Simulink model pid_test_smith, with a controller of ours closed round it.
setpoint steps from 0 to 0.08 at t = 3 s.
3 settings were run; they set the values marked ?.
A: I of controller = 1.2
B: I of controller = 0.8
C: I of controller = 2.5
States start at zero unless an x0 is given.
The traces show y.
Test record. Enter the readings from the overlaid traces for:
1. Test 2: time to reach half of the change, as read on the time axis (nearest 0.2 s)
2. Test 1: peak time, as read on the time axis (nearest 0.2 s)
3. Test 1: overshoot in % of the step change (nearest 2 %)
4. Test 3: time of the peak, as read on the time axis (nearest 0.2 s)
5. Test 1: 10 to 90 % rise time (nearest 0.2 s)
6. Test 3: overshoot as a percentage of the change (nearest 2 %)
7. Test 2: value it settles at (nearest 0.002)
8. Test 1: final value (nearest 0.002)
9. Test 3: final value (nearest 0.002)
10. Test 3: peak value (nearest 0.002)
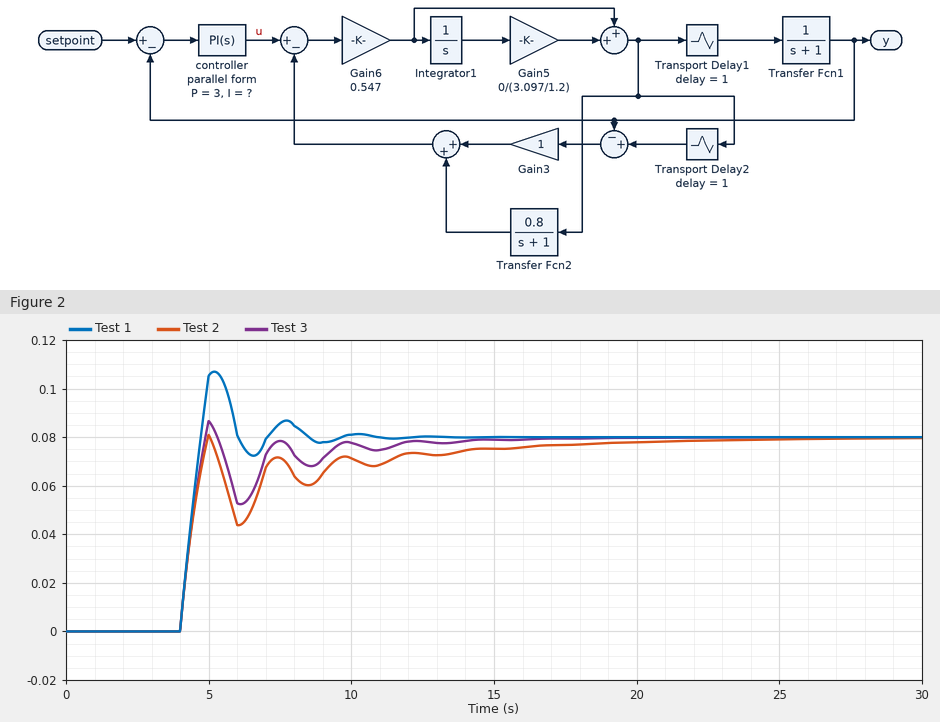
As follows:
4.4 s
5.2 s
34 %
5.0 s
0.6 s
8 %
0.080
0.080
0.080
0.086
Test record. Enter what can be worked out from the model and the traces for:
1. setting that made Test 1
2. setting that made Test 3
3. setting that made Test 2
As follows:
C
A
B
